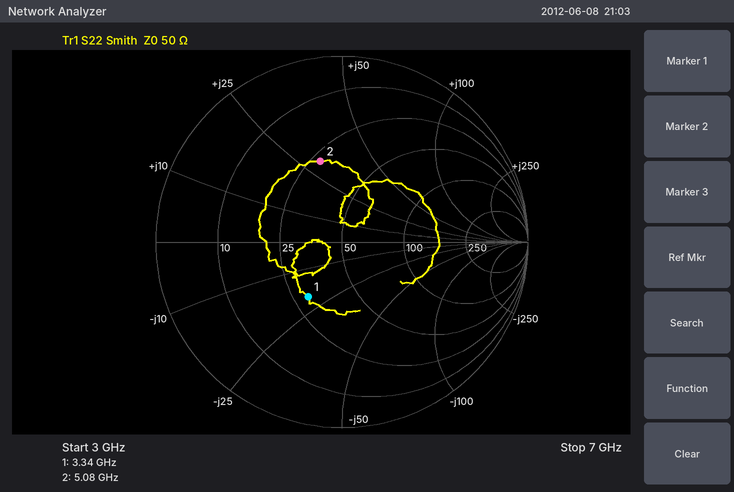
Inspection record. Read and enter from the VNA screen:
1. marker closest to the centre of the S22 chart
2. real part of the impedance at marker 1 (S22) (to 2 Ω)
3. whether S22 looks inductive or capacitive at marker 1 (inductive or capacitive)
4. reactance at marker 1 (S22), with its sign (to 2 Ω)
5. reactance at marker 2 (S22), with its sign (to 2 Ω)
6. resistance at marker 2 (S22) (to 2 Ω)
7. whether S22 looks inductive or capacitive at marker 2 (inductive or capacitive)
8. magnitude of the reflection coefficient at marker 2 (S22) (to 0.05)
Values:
marker 1
30 Ω
capacitive
-20 Ω
+30 Ω
28 Ω
inductive
0.45
